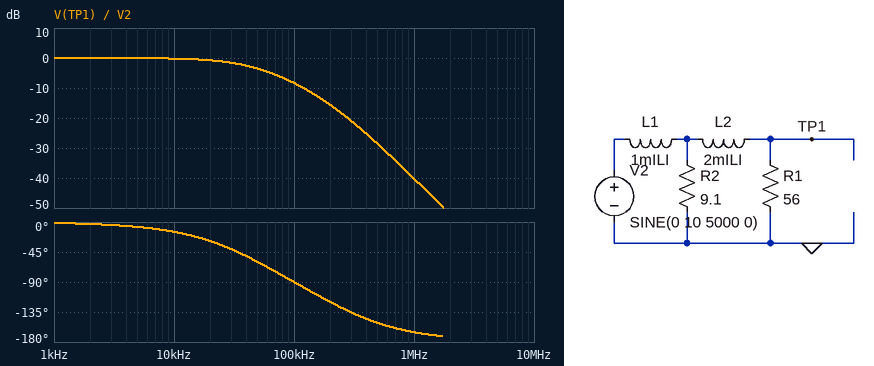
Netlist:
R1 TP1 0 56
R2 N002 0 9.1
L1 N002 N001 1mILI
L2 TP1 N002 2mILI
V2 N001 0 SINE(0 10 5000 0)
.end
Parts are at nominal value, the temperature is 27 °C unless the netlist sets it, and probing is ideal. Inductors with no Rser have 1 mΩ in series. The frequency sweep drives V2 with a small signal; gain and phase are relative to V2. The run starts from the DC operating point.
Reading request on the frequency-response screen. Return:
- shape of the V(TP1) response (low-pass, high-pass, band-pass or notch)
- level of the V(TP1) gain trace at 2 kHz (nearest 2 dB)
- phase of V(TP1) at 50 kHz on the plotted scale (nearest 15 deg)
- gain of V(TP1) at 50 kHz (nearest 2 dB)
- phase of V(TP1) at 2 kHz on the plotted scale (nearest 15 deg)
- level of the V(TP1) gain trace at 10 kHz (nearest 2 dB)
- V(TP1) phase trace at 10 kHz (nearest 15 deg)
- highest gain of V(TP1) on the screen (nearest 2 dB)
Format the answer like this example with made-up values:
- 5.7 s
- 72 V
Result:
- low-pass
- 0 dB
- -60 deg
- -4 dB
- 0 deg
- 0 dB
- -15 deg
- 0 dB
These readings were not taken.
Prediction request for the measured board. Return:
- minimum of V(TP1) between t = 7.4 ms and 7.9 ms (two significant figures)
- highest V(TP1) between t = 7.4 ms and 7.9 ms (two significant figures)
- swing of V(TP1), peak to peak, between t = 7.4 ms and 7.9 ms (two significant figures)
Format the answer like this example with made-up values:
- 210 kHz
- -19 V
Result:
- -9.9 V
- 9.9 V
- 20 V
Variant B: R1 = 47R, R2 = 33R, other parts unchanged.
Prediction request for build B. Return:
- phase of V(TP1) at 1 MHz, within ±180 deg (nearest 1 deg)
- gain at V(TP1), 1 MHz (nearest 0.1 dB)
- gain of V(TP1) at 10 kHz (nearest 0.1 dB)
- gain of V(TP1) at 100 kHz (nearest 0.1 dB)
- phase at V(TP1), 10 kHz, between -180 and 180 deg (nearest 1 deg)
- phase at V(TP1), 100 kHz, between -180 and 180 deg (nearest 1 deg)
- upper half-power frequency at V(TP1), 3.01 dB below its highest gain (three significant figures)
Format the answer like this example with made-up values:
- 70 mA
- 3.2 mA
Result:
- -155 deg
- -30.9 dB
- -0.1 dB
- -4.3 dB
- -9 deg
- -66 deg
- 77.5 kHz
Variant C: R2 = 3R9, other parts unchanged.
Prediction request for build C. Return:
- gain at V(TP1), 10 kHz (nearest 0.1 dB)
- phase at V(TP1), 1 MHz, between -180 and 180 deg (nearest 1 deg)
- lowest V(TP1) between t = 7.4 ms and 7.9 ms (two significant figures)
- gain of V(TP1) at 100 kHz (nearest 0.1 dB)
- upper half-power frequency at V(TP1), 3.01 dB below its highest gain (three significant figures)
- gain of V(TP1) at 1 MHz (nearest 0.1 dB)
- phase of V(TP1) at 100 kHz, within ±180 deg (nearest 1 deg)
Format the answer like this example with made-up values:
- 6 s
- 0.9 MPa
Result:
- -0.8 dB
- -168 deg
- -9.8 V
- -14.2 dB
- 22.3 kHz
- -47.5 dB
- -105 deg
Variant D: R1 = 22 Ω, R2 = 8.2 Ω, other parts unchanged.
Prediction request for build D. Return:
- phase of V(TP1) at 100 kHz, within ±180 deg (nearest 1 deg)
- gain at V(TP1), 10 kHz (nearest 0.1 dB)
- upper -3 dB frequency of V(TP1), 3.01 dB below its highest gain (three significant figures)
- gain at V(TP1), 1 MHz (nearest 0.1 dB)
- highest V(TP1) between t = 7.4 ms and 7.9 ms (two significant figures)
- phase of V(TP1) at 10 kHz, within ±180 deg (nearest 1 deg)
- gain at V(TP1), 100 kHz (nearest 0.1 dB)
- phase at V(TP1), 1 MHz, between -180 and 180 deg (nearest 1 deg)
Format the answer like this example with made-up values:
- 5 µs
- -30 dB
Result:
- -114 deg
- -0.5 dB
- 28.9 kHz
- -49.1 dB
- 9.9 V
- -23 deg
- -13.1 dB
- -172 deg
